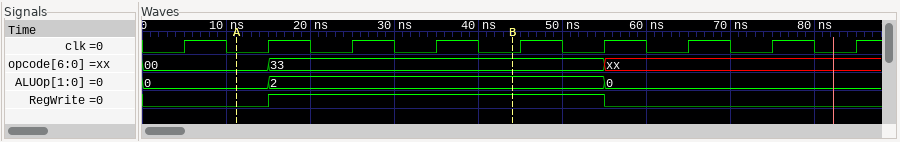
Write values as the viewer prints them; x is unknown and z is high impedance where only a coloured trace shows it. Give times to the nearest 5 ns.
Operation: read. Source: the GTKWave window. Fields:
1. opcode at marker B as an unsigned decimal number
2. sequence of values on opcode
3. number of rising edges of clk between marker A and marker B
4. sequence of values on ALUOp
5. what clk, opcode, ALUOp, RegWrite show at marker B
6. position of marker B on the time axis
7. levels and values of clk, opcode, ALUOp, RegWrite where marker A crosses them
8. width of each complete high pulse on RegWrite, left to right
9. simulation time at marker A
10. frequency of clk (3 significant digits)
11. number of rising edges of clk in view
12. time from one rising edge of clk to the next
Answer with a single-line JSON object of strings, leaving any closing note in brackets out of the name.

{"opcode at marker B as an unsigned decimal number": "51", "sequence of values on opcode": "00, 33, xx", "number of rising edges of clk between marker A and marker B": "3", "sequence of values on ALUOp": "0, 2, 0", "what clk, opcode, ALUOp, RegWrite show at marker B": "clk=0, opcode=33, ALUOp=2, RegWrite=1", "position of marker B on the time axis": "45 ns", "levels and values of clk, opcode, ALUOp, RegWrite where marker A crosses them": "clk=0, opcode=00, ALUOp=0, RegWrite=0", "width of each complete high pulse on RegWrite, left to right": "40 ns", "simulation time at marker A": "10 ns", "frequency of clk": "100 MHz", "number of rising edges of clk in view": "9", "time from one rising edge of clk to the next": "10 ns"}
